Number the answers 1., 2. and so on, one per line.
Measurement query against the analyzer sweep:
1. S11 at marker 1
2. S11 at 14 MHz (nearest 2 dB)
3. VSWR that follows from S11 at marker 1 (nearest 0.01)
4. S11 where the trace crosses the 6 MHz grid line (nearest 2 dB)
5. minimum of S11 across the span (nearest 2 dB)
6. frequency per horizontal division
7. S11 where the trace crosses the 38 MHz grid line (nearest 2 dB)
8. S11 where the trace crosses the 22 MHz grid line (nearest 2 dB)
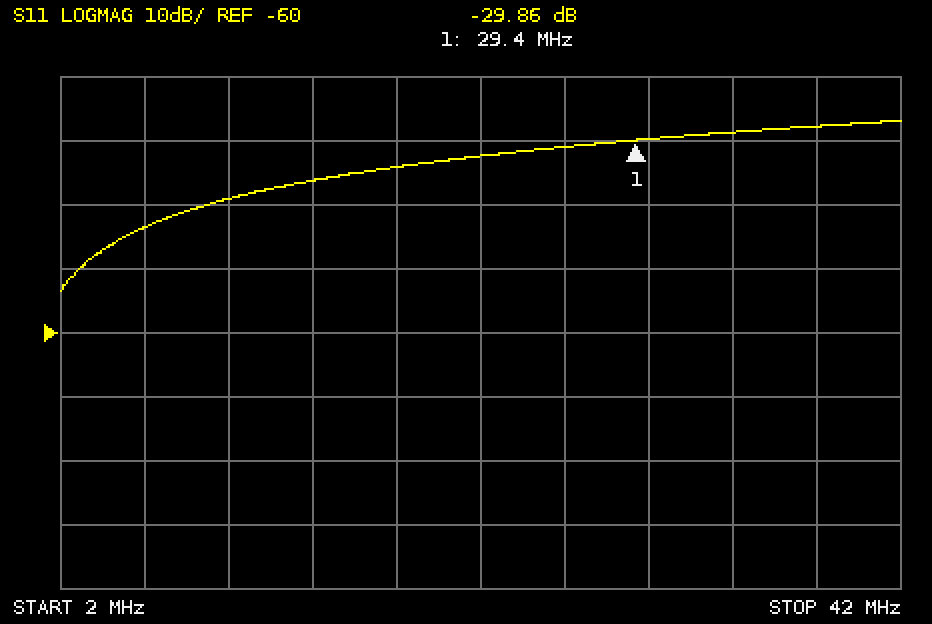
1. -29.86 dB
2. -36 dB
3. 1.07
4. -44 dB
5. -54 dB
6. 4 MHz
7. -28 dB
8. -32 dB
